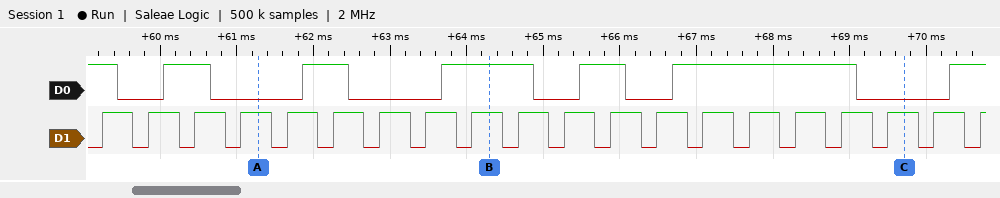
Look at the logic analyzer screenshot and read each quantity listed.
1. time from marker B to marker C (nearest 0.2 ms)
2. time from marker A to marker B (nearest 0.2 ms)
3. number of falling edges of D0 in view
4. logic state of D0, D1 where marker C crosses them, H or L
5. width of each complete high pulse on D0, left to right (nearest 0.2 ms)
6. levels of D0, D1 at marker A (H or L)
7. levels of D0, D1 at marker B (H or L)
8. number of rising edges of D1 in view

5.4 ms
3 ms
6
D0=L, D1=H
0.6 ms, 0.6 ms, 1.2 ms, 0.6 ms, 2.4 ms
D0=L, D1=H
D0=H, D1=H
20
